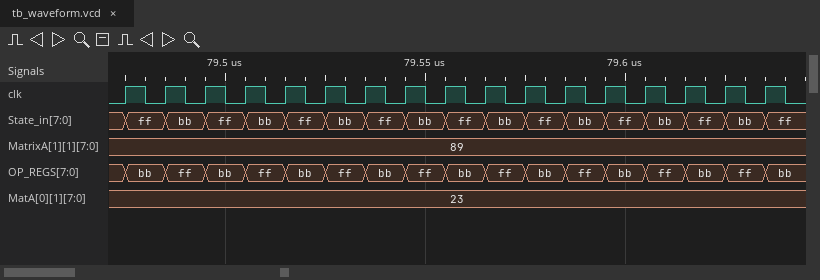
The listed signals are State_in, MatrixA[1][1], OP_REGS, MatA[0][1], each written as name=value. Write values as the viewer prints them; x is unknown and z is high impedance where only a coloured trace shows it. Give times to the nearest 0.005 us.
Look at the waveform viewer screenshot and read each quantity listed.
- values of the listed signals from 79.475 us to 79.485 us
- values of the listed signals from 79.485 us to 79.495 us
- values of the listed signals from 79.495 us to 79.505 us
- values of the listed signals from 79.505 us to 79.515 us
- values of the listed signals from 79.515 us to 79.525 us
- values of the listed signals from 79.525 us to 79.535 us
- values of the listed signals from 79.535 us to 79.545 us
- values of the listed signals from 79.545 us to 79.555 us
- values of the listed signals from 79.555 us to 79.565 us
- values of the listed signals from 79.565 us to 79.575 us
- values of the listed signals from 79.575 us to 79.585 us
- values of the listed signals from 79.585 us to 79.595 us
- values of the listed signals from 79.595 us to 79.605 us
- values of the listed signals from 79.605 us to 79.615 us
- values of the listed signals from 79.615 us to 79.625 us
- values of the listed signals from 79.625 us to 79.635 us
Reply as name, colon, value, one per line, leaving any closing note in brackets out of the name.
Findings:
values of the listed signals from 79.475 us to 79.485 us: State_in=ff, MatrixA[1][1]=89, OP_REGS=bb, MatA[0][1]=23
values of the listed signals from 79.485 us to 79.495 us: State_in=bb, MatrixA[1][1]=89, OP_REGS=ff, MatA[0][1]=23
values of the listed signals from 79.495 us to 79.505 us: State_in=ff, MatrixA[1][1]=89, OP_REGS=bb, MatA[0][1]=23
values of the listed signals from 79.505 us to 79.515 us: State_in=bb, MatrixA[1][1]=89, OP_REGS=ff, MatA[0][1]=23
values of the listed signals from 79.515 us to 79.525 us: State_in=ff, MatrixA[1][1]=89, OP_REGS=bb, MatA[0][1]=23
values of the listed signals from 79.525 us to 79.535 us: State_in=bb, MatrixA[1][1]=89, OP_REGS=ff, MatA[0][1]=23
values of the listed signals from 79.535 us to 79.545 us: State_in=ff, MatrixA[1][1]=89, OP_REGS=bb, MatA[0][1]=23
values of the listed signals from 79.545 us to 79.555 us: State_in=bb, MatrixA[1][1]=89, OP_REGS=ff, MatA[0][1]=23
values of the listed signals from 79.555 us to 79.565 us: State_in=ff, MatrixA[1][1]=89, OP_REGS=bb, MatA[0][1]=23
values of the listed signals from 79.565 us to 79.575 us: State_in=bb, MatrixA[1][1]=89, OP_REGS=ff, MatA[0][1]=23
values of the listed signals from 79.575 us to 79.585 us: State_in=ff, MatrixA[1][1]=89, OP_REGS=bb, MatA[0][1]=23
values of the listed signals from 79.585 us to 79.595 us: State_in=bb, MatrixA[1][1]=89, OP_REGS=ff, MatA[0][1]=23
values of the listed signals from 79.595 us to 79.605 us: State_in=ff, MatrixA[1][1]=89, OP_REGS=bb, MatA[0][1]=23
values of the listed signals from 79.605 us to 79.615 us: State_in=bb, MatrixA[1][1]=89, OP_REGS=ff, MatA[0][1]=23
values of the listed signals from 79.615 us to 79.625 us: State_in=ff, MatrixA[1][1]=89, OP_REGS=bb, MatA[0][1]=23
values of the listed signals from 79.625 us to 79.635 us: State_in=bb, MatrixA[1][1]=89, OP_REGS=ff, MatA[0][1]=23
